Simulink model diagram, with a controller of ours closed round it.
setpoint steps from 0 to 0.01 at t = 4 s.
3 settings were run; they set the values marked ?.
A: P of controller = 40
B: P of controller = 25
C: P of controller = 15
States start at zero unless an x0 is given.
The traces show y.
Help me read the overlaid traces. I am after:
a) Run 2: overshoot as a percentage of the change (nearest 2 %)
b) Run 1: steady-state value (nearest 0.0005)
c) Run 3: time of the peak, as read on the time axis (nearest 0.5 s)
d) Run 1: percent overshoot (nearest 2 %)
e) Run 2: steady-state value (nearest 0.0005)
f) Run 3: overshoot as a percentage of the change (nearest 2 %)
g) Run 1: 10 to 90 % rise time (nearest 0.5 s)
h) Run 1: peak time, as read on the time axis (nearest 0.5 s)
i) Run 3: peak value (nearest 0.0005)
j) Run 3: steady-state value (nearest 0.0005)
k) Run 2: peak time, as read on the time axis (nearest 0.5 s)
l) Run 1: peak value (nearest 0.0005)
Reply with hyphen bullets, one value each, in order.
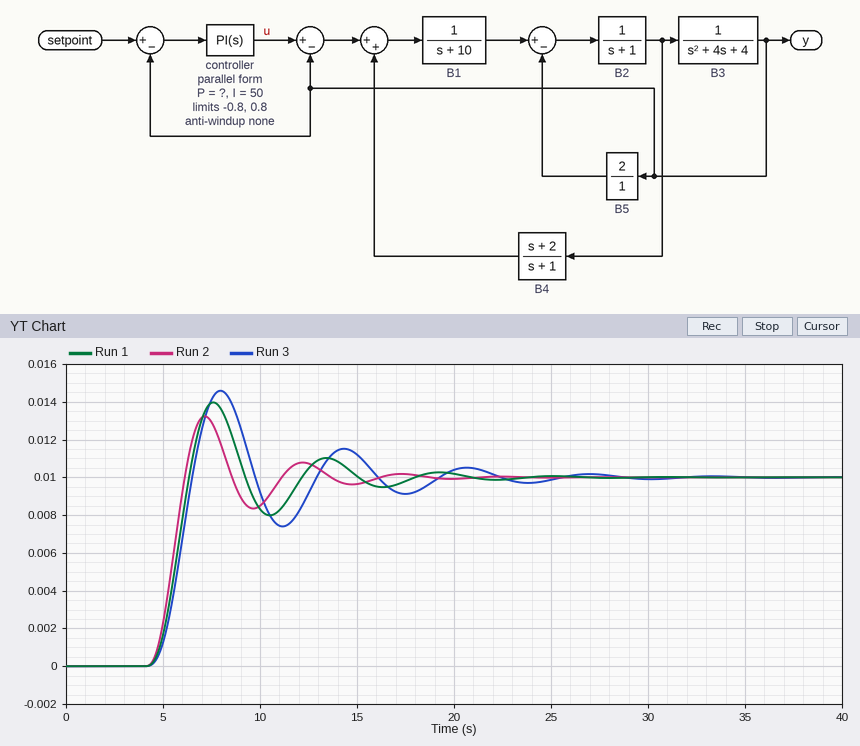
- 32 %
- 0.0100
- 8.0 s
- 40 %
- 0.0100
- 46 %
- 1.5 s
- 7.5 s
- 0.0145
- 0.0100
- 7.0 s
- 0.0140
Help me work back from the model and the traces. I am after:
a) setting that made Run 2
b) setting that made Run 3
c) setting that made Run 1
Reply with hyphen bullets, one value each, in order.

- A
- C
- B
